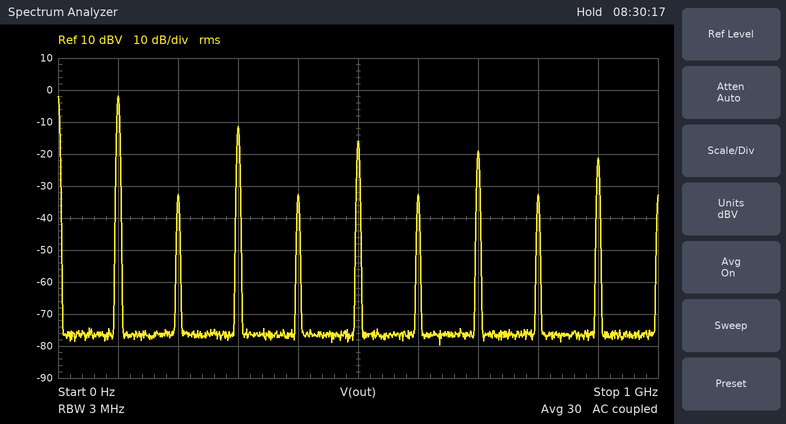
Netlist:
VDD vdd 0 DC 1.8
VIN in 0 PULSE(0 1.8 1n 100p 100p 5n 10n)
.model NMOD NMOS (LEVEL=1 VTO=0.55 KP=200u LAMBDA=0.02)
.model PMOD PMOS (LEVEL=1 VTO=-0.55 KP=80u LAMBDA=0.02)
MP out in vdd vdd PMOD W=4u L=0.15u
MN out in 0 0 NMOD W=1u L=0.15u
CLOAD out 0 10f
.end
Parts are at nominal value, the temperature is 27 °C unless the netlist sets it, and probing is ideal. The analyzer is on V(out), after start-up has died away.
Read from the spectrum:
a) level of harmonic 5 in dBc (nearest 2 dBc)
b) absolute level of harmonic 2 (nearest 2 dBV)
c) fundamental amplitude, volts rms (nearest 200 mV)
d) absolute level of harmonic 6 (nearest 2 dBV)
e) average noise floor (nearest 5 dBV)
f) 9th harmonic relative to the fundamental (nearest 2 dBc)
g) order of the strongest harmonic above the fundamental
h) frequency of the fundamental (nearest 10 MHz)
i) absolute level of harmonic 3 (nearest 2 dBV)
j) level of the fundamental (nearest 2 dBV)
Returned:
-14 dBc
-32 dBV
800 mV
-32 dBV
-75 dBV
-20 dBc
3
100 MHz
-12 dBV
-2 dBV
